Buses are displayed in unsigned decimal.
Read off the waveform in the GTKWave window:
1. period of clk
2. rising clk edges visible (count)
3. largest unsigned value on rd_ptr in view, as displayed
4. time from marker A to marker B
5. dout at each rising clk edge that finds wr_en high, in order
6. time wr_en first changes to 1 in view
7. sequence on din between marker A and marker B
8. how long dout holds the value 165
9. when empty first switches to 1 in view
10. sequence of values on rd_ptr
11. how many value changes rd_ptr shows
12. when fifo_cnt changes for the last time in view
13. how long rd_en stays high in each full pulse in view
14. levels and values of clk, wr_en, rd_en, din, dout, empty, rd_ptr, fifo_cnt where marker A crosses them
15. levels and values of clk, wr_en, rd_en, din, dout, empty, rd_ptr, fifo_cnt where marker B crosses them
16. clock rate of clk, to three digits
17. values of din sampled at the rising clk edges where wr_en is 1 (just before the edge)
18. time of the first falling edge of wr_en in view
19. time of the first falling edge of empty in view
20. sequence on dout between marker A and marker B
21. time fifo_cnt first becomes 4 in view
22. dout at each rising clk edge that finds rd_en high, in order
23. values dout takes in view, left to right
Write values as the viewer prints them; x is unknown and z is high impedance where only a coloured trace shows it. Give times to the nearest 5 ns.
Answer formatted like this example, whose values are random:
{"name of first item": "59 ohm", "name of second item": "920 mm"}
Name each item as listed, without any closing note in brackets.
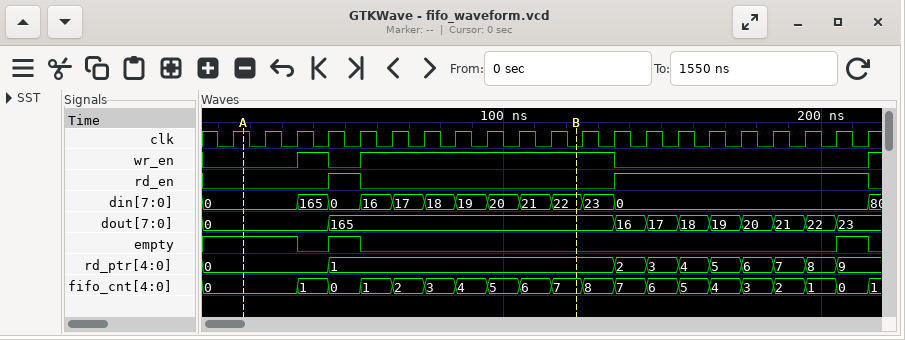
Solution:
{"period of clk": "10 ns", "rising clk edges visible": "21", "largest unsigned value on rd_ptr in view, as displayed": "9", "time from marker A to marker B": "105 ns", "dout at each rising clk edge that finds wr_en high, in order": "0, 165, 165, 165, 165, 165, 165, 165, 165", "time wr_en first changes to 1 in view": "35 ns", "sequence on din between marker A and marker B": "0, 165, 0, 16, 17, 18, 19, 20, 21, 22", "how long dout holds the value 165": "90 ns", "when empty first switches to 1 in view": "45 ns", "sequence of values on rd_ptr": "0, 1, 2, 3, 4, 5, 6, 7, 8, 9", "how many value changes rd_ptr shows": "9", "when fifo_cnt changes for the last time in view": "215 ns", "how long rd_en stays high in each full pulse in view": "10 ns, 80 ns", "levels and values of clk, wr_en, rd_en, din, dout, empty, rd_ptr, fifo_cnt where marker A crosses them": "clk=1, wr_en=0, rd_en=0, din=0, dout=0, empty=1, rd_ptr=0, fifo_cnt=0", "levels and values of clk, wr_en, rd_en, din, dout, empty, rd_ptr, fifo_cnt where marker B crosses them": "clk=0, wr_en=1, rd_en=0, din=22, dout=165, empty=0, rd_ptr=1, fifo_cnt=7", "clock rate of clk, to three digits": "100 MHz", "values of din sampled at the rising clk edges where wr_en is 1": "165, 16, 17, 18, 19, 20, 21, 22, 23", "time of the first falling edge of wr_en in view": "45 ns", "time of the first falling edge of empty in view": "35 ns", "sequence on dout between marker A and marker B": "0, 165", "time fifo_cnt first becomes 4 in view": "85 ns", "dout at each rising clk edge that finds rd_en high, in order": "165, 16, 17, 18, 19, 20, 21, 22, 23", "values dout takes in view, left to right": "0, 165, 16, 17, 18, 19, 20, 21, 22, 23"}
